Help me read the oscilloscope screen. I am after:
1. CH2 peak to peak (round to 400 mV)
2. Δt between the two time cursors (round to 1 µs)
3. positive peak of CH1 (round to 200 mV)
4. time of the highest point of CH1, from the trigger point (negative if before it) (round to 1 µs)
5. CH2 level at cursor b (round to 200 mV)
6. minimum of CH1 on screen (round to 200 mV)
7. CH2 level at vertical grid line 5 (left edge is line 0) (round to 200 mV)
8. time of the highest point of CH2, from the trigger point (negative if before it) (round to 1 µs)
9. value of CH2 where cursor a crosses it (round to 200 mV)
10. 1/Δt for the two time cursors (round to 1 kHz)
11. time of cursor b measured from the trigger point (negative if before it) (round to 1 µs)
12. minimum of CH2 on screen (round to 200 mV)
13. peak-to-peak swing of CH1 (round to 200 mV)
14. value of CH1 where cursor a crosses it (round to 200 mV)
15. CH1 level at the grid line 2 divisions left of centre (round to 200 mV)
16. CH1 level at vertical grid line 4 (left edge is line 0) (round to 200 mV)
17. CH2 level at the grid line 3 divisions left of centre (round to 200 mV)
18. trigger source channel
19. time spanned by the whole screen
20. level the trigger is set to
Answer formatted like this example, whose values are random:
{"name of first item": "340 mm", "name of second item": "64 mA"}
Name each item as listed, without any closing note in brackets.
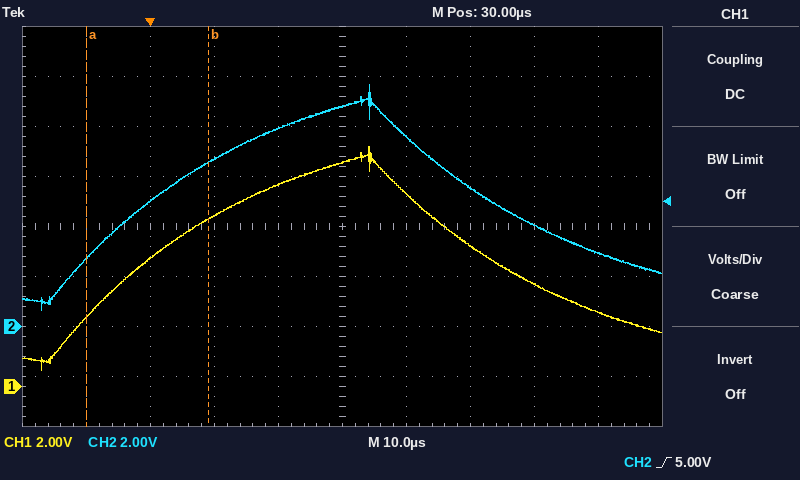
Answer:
{"CH2 peak to peak": "9.2 V", "Δt between the two time cursors": "19 µs", "positive peak of CH1": "9.6 V", "time of the highest point of CH1, from the trigger point (negative if before it)": "+34 µs", "CH2 level at cursor b": "6.6 V", "minimum of CH1 on screen": "600 mV", "CH2 level at vertical grid line 5 (left edge is line 0)": "8.8 V", "time of the highest point of CH2, from the trigger point (negative if before it)": "+34 µs", "value of CH2 where cursor a crosses it": "2.8 V", "1/Δt for the two time cursors": "53 kHz", "time of cursor b measured from the trigger point (negative if before it)": "+9 µs", "minimum of CH2 on screen": "600 mV", "peak-to-peak swing of CH1": "9.0 V", "value of CH1 where cursor a crosses it": "2.8 V", "CH1 level at the grid line 2 divisions left of centre": "6.8 V", "CH1 level at vertical grid line 4 (left edge is line 0)": "8.0 V", "CH2 level at the grid line 3 divisions left of centre": "5.0 V", "trigger source channel": "CH2", "time spanned by the whole screen": "100 µs", "level the trigger is set to": "5.00 V"}
